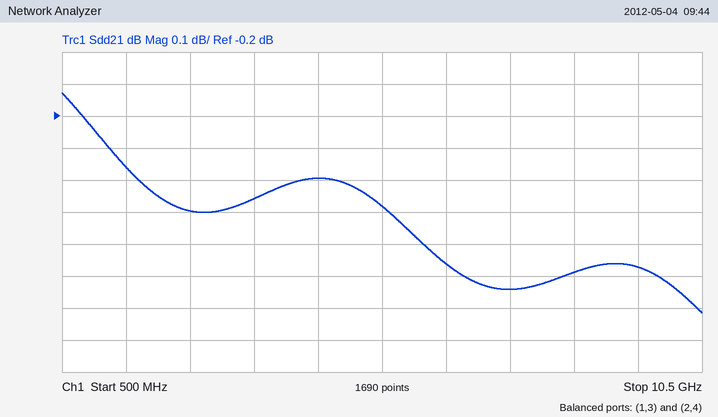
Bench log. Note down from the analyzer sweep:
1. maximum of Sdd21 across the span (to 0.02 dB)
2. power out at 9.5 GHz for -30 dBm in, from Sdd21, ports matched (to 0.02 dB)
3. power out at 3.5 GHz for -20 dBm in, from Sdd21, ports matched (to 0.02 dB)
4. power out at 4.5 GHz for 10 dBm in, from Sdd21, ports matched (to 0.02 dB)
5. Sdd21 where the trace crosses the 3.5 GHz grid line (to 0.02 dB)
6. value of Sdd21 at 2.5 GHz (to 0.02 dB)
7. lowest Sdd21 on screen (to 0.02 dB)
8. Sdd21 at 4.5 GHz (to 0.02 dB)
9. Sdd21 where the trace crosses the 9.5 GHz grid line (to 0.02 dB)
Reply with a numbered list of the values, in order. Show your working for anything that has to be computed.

1. -0.12 dB
2. -30 dBm + (-0.68 dB) = -30.68 dBm
3. -20 dBm + (-0.46 dB) = -20.46 dBm
4. 10 dBm + (-0.40 dB) = 9.60 dBm
5. -0.46 dB
6. -0.50 dB
7. -0.82 dB
8. -0.40 dB
9. -0.68 dB
